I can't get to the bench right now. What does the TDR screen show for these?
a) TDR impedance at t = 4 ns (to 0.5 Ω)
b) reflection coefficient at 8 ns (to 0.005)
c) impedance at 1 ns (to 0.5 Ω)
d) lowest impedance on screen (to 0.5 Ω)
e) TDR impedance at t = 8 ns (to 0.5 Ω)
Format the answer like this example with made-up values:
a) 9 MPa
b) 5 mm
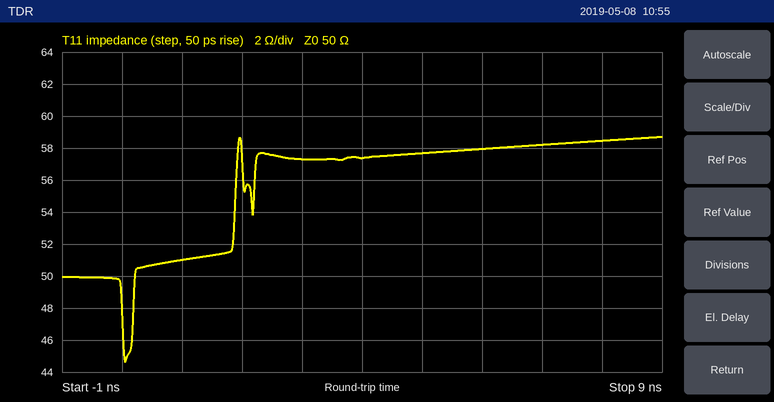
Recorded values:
a) 57.5 Ω
b) +0.080
c) 51.0 Ω
d) 44.5 Ω
e) 58.5 Ω
